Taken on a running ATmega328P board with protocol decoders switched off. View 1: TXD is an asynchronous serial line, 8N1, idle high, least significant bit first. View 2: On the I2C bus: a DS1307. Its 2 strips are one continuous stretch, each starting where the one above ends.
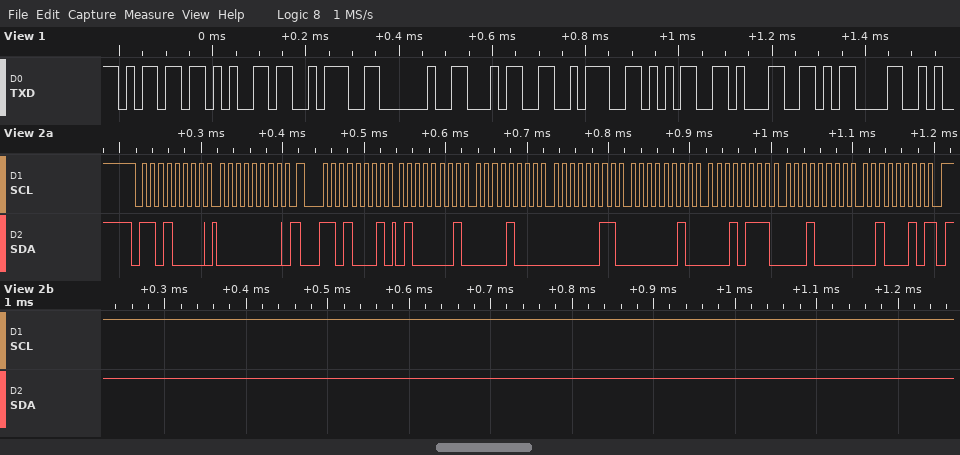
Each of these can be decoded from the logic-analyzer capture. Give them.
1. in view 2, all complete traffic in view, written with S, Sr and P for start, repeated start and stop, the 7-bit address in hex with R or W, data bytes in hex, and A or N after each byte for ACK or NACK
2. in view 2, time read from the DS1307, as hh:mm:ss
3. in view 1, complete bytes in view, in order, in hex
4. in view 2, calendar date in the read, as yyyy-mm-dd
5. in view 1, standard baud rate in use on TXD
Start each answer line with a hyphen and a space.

- S 68W A 00 A Sr 68R A 41 A 08 A 03 A 02 A 17 A 10 A 22 N P
- 03:08:41
- 6D 65 3A 20 34 3A 35 31 0D
- 2022-10-17
- 57600 baud
